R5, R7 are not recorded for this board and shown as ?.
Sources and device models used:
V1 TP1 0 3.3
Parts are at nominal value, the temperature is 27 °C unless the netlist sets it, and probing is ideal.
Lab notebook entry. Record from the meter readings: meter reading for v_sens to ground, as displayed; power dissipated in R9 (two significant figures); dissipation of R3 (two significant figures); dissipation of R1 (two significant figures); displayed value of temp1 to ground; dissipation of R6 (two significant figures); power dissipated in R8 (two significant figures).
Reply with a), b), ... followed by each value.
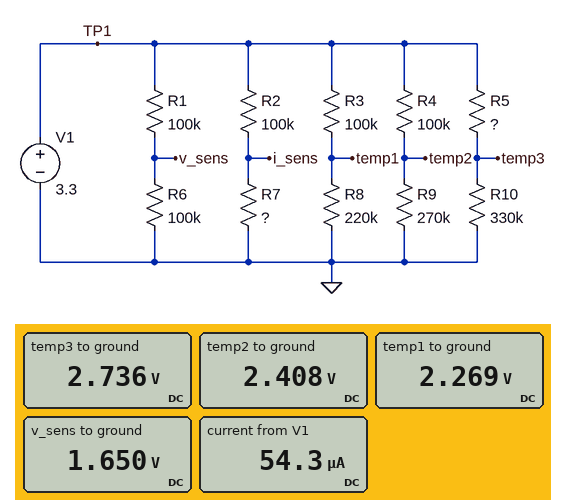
a) 1.650 V
b) 21 µW
c) 11 µW
d) 27 µW
e) 2.269 V
f) 27 µW
g) 23 µW
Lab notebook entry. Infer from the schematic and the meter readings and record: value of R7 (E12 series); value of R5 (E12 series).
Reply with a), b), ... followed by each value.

a) 220 kΩ
b) 68 kΩ
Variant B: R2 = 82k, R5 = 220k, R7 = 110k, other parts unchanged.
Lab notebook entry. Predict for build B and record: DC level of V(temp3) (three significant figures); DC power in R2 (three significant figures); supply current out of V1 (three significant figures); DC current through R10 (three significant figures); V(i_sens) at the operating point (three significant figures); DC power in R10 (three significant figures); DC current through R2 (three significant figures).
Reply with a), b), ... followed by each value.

a) 1.98 V
b) 24.2 µW
c) 58.9 µA
d) 6.00 µA
e) 1.89 V
f) 11.9 µW
g) 17.2 µA
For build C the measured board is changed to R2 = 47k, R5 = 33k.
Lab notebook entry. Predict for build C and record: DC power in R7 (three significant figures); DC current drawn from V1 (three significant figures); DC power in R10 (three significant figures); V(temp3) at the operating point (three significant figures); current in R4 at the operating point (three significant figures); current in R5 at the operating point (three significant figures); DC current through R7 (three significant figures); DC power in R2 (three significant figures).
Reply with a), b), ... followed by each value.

a) 33.6 µW
b) 57.2 µA
c) 27.3 µW
d) 3.00 V
e) 8.92 µA
f) 9.09 µA
g) 12.4 µA
h) 7.18 µW
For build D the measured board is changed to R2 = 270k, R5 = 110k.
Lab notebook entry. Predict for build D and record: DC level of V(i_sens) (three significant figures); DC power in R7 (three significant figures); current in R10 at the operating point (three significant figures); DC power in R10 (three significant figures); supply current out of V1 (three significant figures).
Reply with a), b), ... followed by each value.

a) 1.48 V
b) 9.98 µW
c) 7.50 µA
d) 18.6 µW
e) 50.0 µA
